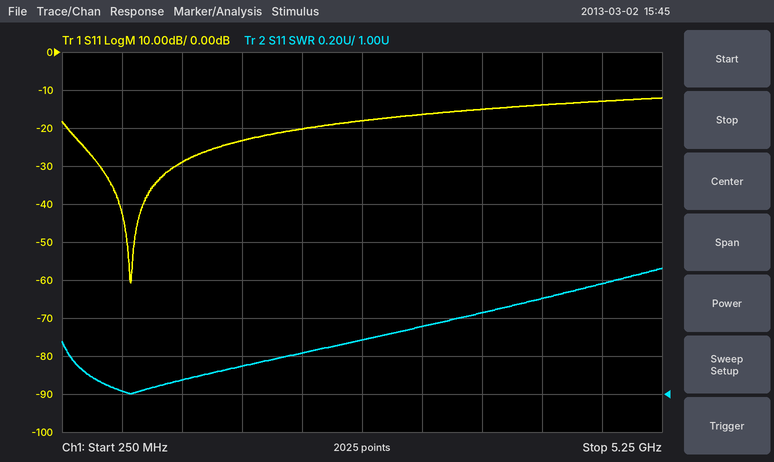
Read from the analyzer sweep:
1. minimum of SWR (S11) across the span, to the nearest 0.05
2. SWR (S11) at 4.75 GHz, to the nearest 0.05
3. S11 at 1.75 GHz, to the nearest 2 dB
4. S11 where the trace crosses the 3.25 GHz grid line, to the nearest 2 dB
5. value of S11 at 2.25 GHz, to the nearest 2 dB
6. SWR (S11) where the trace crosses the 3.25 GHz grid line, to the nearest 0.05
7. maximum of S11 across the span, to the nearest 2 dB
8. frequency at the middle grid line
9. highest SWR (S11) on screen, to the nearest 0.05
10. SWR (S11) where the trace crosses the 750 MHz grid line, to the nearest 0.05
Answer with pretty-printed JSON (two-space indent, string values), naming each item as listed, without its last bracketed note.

{
  "minimum of SWR (S11) across the span, to the nearest 0.05": "1.00",
  "SWR (S11) at 4.75 GHz, to the nearest 0.05": "1.60",
  "S11 at 1.75 GHz, to the nearest 2 dB": "-24 dB",
  "S11 where the trace crosses the 3.25 GHz grid line, to the nearest 2 dB": "-16 dB",
  "value of S11 at 2.25 GHz, to the nearest 2 dB": "-20 dB",
  "SWR (S11) where the trace crosses the 3.25 GHz grid line, to the nearest 0.05": "1.35",
  "maximum of S11 across the span, to the nearest 2 dB": "-12 dB",
  "frequency at the middle grid line": "2.75 GHz",
  "highest SWR (S11) on screen, to the nearest 0.05": "1.65",
  "SWR (S11) where the trace crosses the 750 MHz grid line, to the nearest 0.05": "1.00"
}
